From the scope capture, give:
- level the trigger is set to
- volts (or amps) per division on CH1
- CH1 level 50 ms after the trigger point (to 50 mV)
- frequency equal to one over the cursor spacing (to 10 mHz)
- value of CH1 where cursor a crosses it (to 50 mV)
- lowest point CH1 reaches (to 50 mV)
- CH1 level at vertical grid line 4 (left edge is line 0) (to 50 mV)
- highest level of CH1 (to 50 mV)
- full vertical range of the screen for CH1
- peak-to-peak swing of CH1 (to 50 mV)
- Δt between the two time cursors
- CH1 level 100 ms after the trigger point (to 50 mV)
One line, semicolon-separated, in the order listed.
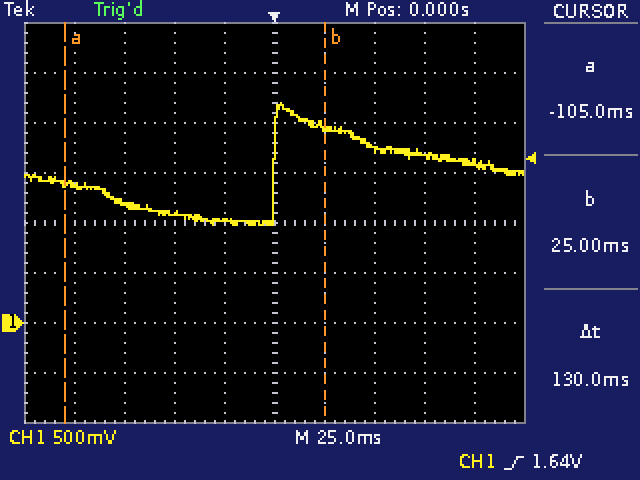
1.64 V; 500 mV; 1.75 V; 7.69 Hz; 1.40 V; 1.00 V; 1.05 V; 2.20 V; 4 V; 1.20 V; 130 ms; 1.60 V
